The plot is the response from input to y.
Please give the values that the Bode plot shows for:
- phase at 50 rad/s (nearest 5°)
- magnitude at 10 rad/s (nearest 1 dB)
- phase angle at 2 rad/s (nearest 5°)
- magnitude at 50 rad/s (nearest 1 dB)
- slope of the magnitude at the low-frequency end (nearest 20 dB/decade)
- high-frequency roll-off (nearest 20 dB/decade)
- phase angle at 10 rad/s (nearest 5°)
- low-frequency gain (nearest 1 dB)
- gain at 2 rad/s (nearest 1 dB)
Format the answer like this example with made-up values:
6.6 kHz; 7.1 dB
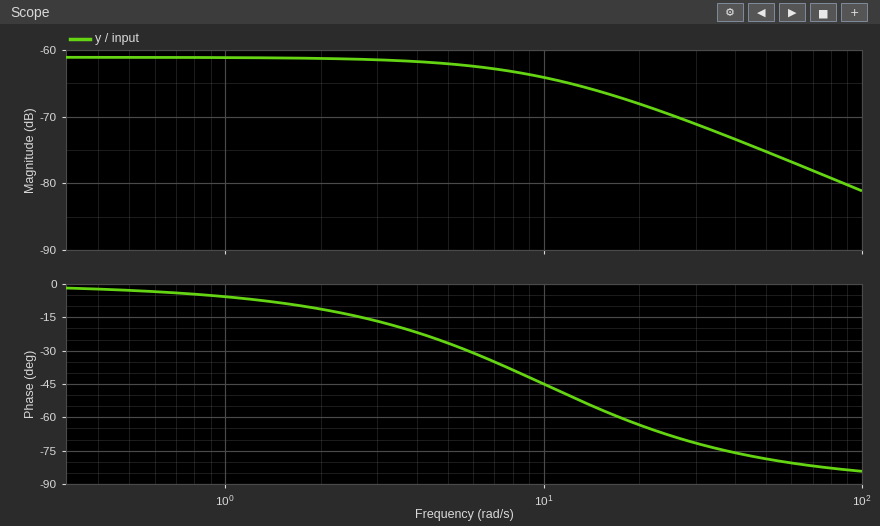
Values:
-80°; -64 dB; -10°; -75 dB; 0 dB/decade; -20 dB/decade; -45°; -61 dB; -61 dB
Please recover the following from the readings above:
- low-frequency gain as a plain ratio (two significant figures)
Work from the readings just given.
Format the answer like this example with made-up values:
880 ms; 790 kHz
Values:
0.00089
